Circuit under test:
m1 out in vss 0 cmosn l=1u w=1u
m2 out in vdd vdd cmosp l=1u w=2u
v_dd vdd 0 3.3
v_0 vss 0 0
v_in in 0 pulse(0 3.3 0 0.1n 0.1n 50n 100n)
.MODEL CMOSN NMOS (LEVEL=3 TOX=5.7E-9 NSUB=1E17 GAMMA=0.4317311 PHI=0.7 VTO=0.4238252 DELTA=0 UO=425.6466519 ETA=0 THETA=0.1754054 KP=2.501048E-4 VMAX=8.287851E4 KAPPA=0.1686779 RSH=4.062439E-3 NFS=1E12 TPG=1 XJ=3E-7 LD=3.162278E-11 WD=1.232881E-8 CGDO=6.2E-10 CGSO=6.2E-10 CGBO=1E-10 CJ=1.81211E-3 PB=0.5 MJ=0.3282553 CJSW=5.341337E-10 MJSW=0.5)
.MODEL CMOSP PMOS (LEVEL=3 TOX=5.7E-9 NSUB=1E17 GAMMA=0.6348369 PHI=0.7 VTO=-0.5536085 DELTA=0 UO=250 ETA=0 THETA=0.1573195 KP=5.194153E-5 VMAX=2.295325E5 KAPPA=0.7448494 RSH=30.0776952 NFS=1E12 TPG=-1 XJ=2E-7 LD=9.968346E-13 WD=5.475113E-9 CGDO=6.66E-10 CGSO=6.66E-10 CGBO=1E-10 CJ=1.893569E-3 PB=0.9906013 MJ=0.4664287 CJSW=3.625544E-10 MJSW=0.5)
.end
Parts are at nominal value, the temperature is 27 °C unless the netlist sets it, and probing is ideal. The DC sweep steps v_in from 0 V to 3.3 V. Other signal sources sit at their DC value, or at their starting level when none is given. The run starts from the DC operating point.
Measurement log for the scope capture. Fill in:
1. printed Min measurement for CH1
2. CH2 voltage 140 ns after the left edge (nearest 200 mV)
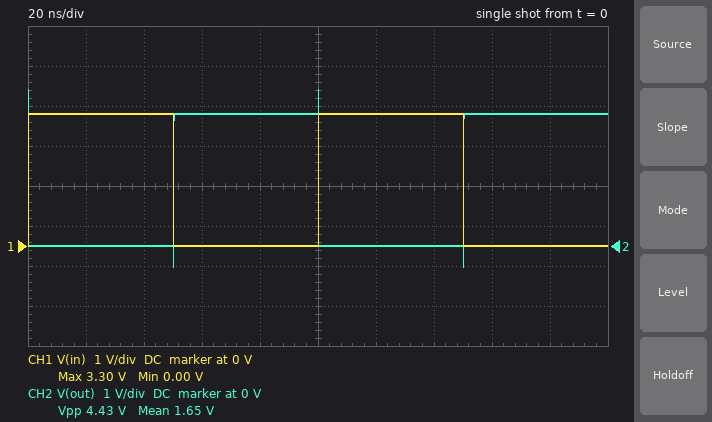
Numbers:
0.00 V
0 V
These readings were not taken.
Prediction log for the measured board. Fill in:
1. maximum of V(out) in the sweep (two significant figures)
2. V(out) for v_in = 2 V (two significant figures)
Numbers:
3.3 V
81 mV
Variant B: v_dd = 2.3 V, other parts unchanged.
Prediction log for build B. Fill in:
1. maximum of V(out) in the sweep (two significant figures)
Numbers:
2.3 V
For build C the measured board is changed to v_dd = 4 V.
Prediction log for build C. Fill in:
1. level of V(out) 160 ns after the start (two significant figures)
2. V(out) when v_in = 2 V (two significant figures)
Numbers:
4.0 V
300 mV
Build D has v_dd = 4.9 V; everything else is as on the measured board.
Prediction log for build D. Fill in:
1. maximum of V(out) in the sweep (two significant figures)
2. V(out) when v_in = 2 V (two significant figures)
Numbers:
4.9 V
3.3 V
